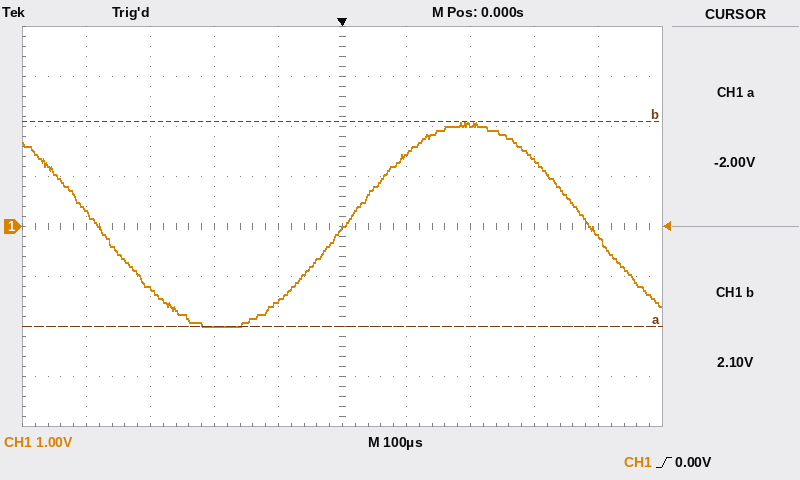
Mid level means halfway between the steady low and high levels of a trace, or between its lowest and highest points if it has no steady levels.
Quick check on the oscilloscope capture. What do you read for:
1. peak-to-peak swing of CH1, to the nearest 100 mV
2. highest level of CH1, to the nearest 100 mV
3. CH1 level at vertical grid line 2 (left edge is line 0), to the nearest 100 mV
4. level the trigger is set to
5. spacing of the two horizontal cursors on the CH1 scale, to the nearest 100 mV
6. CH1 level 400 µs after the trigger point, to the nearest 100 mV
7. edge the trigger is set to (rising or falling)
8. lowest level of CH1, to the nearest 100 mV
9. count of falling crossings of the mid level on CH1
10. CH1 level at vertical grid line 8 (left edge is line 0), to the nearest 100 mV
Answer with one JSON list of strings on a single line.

["4.1 V", "2.1 V", "-1.2 V", "0.00 V", "4.1 V", "-200 mV", "rising", "-2.0 V", "2", "1.3 V"]
